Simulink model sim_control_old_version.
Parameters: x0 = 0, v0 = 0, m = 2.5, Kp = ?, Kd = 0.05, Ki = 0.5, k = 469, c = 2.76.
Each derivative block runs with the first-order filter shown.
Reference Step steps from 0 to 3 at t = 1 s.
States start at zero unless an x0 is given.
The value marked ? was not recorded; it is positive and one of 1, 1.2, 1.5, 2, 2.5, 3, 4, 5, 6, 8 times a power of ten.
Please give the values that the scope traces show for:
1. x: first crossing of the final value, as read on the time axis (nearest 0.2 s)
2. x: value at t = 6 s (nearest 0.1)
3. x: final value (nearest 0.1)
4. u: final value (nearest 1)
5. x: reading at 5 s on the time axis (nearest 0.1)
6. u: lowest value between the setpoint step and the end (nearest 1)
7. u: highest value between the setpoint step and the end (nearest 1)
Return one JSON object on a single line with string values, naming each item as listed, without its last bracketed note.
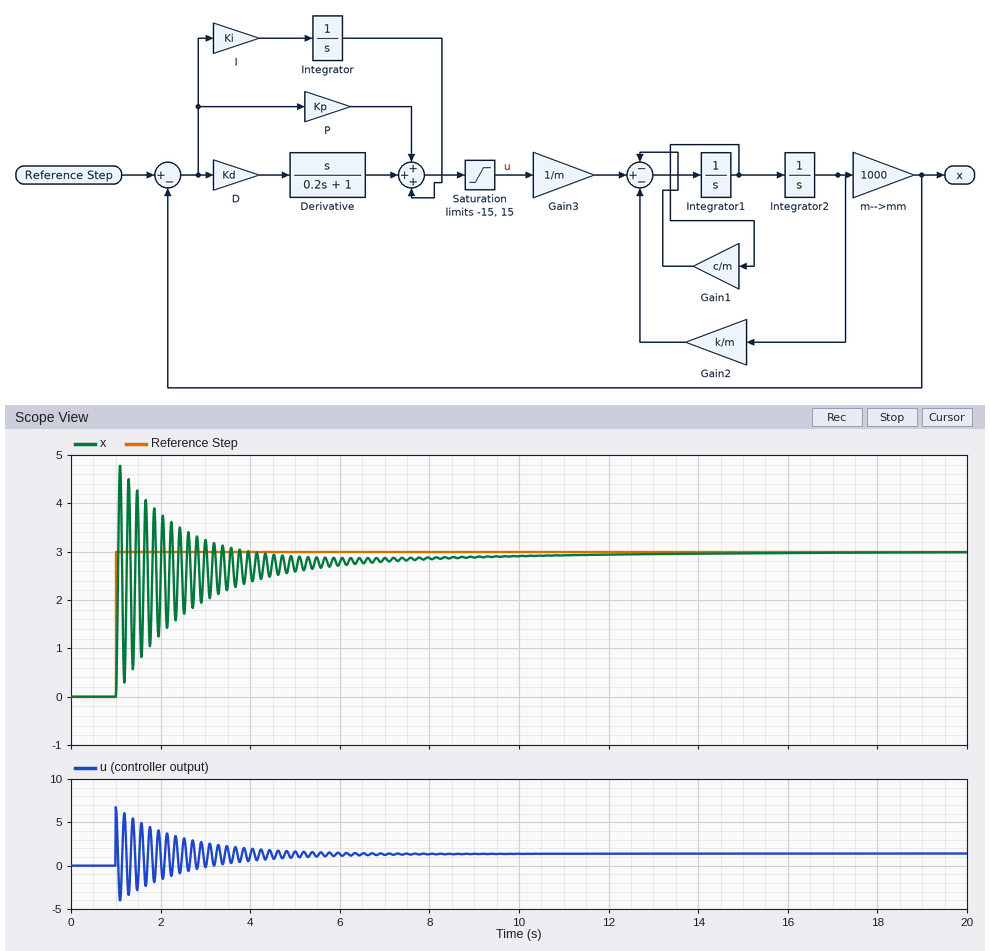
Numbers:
{"x: first crossing of the final value, as read on the time axis": "1.0 s", "x: value at t = 6 s": "2.8", "x: final value": "3.0", "u: final value": "1", "x: reading at 5 s on the time axis": "2.6", "u: lowest value between the setpoint step and the end": "-4", "u: highest value between the setpoint step and the end": "7"}
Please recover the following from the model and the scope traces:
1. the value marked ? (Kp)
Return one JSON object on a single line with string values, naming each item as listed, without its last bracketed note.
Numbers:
{"the value marked ?": "2"}
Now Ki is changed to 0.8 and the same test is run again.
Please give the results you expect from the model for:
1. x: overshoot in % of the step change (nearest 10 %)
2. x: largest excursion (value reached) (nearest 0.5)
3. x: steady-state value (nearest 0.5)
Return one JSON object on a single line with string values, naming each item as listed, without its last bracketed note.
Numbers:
{"x: overshoot in % of the step change": "60 %", "x: largest excursion (value reached)": "5.0", "x: steady-state value": "3.0"}
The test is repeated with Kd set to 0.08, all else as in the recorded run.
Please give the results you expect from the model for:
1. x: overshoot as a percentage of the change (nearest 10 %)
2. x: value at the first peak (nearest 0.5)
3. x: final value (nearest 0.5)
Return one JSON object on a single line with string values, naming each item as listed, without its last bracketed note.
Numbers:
{"x: overshoot as a percentage of the change": "60 %", "x: value at the first peak": "5.0", "x: final value": "3.0"}
